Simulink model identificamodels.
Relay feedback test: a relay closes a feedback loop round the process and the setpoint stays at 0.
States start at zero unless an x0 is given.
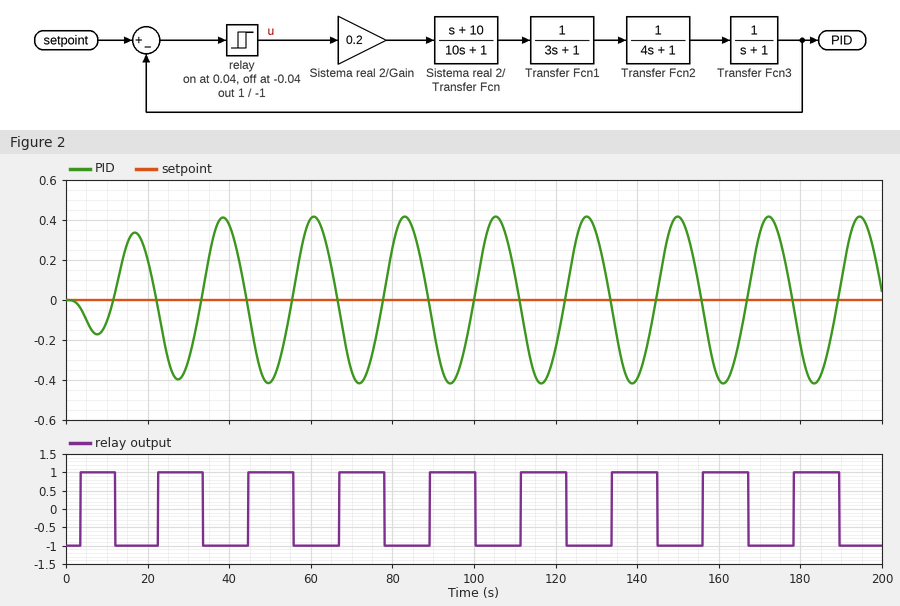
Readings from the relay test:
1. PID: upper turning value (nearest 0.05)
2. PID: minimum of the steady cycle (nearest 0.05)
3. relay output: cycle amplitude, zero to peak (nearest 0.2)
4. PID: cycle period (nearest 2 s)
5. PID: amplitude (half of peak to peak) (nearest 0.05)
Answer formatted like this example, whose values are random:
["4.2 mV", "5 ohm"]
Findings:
["0.40", "-0.40", "1.0", "22 s", "0.40"]
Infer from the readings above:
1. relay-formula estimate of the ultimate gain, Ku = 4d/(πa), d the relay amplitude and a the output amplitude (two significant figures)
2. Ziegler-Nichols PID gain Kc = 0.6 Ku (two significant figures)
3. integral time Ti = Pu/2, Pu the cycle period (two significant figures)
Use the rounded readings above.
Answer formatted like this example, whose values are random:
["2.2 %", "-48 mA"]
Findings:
["3.2", "1.9", "11 s"]
